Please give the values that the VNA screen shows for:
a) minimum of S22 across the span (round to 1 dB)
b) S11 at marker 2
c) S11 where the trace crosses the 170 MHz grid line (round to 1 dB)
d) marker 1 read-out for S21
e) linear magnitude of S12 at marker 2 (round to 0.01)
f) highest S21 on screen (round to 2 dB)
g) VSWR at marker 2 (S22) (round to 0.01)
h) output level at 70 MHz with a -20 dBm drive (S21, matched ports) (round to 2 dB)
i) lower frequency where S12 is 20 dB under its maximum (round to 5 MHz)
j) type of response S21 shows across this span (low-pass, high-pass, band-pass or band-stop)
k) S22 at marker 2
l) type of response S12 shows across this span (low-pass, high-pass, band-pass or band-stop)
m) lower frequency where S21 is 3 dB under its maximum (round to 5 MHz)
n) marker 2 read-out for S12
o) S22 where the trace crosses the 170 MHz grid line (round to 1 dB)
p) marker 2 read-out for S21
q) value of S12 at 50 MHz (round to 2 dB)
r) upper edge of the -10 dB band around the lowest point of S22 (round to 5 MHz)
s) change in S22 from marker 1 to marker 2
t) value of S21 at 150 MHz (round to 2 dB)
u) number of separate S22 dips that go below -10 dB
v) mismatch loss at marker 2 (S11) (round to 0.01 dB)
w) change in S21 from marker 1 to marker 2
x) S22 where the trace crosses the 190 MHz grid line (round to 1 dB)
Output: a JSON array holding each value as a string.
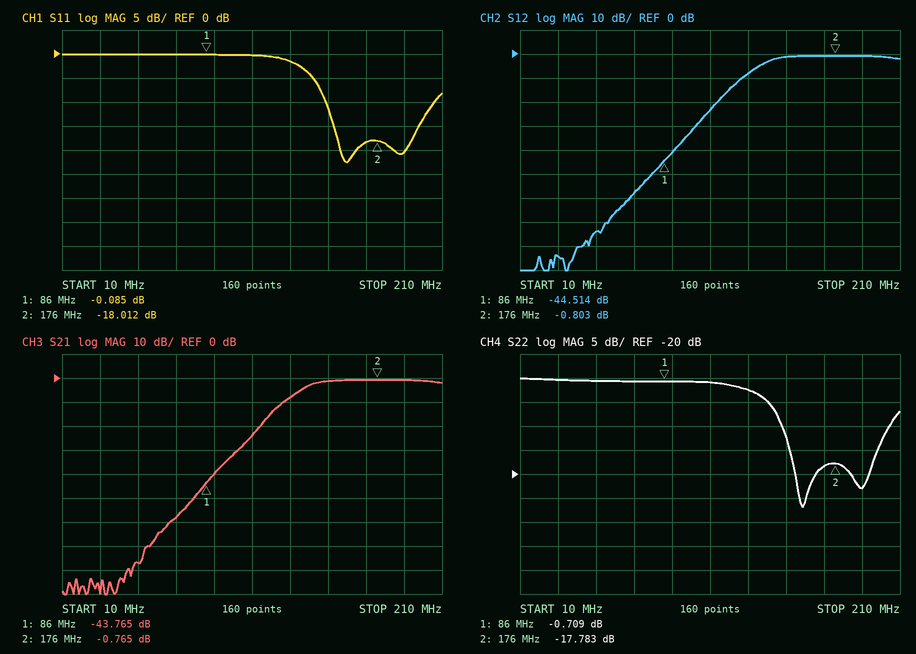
["-27 dB", "-18.012 dB", "-18 dB", "-43.765 dB", "0.91", "0 dB", "1.30", "-78 dBm", "115 MHz", "high-pass", "-17.783 dB", "high-pass", "140 MHz", "-0.803 dB", "-18 dB", "-0.765 dB", "-74 dB", "205 MHz", "-17.074 dB", "-2 dB", "2", "0.07 dB", "43.000 dB", "-23 dB"]
